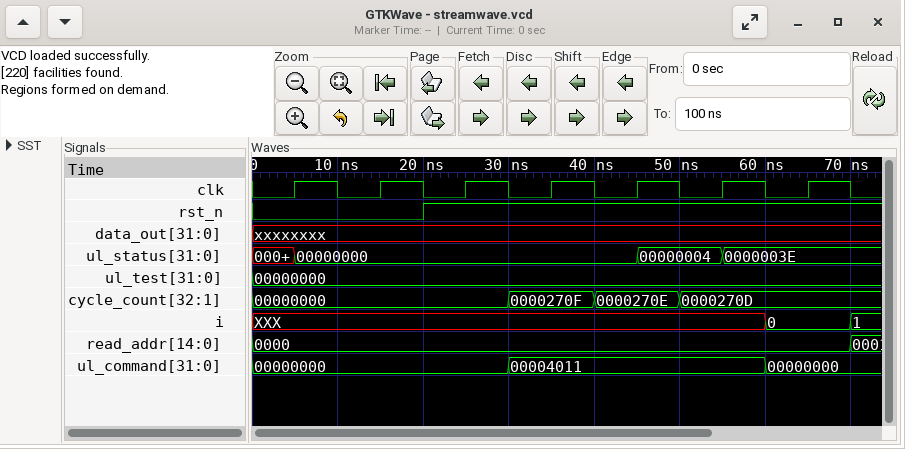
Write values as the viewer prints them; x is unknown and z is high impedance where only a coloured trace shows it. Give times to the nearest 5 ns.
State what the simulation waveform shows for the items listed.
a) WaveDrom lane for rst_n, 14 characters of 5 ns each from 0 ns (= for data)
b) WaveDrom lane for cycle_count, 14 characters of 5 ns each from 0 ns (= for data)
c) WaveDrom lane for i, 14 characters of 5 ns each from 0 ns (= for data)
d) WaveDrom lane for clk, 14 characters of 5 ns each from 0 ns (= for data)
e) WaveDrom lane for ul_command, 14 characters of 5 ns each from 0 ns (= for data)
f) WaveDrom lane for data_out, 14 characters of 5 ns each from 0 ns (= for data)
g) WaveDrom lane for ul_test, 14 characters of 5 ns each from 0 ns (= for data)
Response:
{name: 'rst_n', wave: '0...1.........'}
{name: 'cycle_count', wave: '=.....=.=.=...', data: '00000000 0000270F 0000270E 0000270D'}
{name: 'i', wave: 'x...........=.', data: '0'}
{name: 'clk', wave: '01010101010101'}
{name: 'ul_command', wave: '=.....=.....=.', data: '00000000 00004011 00000000'}
{name: 'data_out', wave: 'x.............'}
{name: 'ul_test', wave: '=.............', data: '00000000'}
